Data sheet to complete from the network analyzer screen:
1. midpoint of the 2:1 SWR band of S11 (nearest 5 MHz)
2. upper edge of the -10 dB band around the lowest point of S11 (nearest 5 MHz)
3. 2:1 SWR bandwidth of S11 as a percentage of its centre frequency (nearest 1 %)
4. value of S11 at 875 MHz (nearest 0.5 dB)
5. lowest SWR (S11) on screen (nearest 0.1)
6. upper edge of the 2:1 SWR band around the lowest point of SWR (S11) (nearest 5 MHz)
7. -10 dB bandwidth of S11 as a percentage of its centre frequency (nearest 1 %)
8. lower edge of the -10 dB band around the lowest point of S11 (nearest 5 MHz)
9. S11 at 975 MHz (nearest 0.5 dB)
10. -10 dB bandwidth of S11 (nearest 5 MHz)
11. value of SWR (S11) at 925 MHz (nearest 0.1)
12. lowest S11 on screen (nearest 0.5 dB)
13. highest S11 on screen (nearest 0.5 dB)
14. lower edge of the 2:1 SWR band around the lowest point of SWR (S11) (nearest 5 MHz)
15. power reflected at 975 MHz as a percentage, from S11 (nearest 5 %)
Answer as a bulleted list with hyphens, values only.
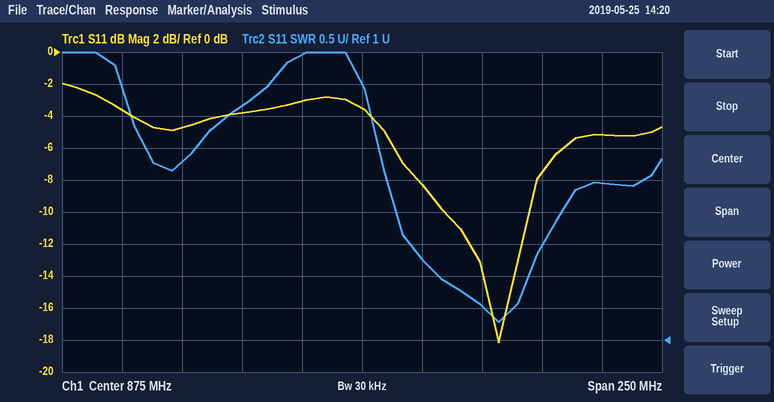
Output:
- 925 MHz
- 945 MHz
- 4 %
- -3.5 dB
- 1.3
- 945 MHz
- 4 %
- 910 MHz
- -5.0 dB
- 35 MHz
- 1.5
- -18.0 dB
- -2.0 dB
- 905 MHz
- 30 %
